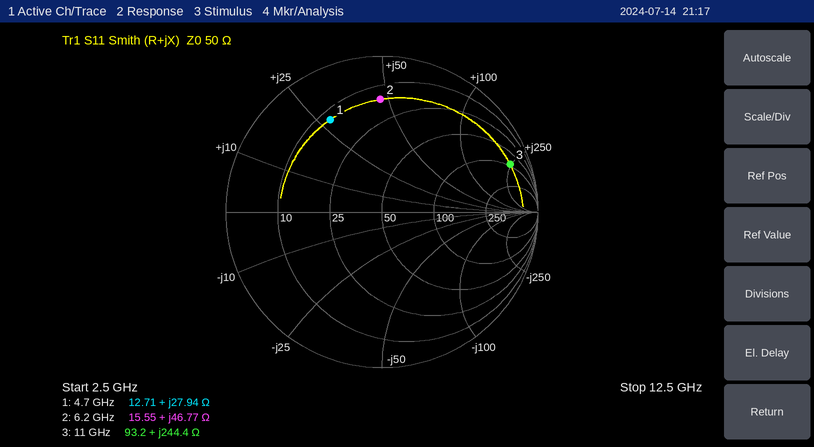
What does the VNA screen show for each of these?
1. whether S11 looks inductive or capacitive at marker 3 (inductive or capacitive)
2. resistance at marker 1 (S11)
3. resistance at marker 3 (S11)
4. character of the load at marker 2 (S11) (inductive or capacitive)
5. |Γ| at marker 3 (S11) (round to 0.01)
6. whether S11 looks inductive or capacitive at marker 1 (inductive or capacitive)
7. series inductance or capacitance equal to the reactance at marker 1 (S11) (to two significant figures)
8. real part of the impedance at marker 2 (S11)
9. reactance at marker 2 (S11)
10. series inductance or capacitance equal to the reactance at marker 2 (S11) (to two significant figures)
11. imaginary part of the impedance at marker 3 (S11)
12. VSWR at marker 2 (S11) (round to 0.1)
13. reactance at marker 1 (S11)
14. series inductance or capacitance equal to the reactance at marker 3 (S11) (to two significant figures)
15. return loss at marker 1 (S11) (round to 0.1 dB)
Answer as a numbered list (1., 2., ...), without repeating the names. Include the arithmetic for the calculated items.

1. inductive
2. 12.71 Ω
3. 93.2 Ω
4. inductive
5. 0.88
6. inductive
7. L = 27.94 Ω/(2π × 4.7 GHz) ≈ 946 pH, so 950 pH to two significant figures
8. 15.55 Ω
9. +46.77 Ω
10. L = 46.77 Ω/(2π × 6.2 GHz) ≈ 1.2 nH
11. +244.4 Ω
12. 6.2
13. +27.94 Ω
14. L = 244.4 Ω/(2π × 11 GHz) ≈ 3.5 nH
15. 3.4 dB
